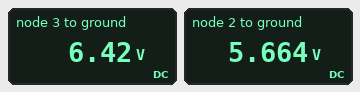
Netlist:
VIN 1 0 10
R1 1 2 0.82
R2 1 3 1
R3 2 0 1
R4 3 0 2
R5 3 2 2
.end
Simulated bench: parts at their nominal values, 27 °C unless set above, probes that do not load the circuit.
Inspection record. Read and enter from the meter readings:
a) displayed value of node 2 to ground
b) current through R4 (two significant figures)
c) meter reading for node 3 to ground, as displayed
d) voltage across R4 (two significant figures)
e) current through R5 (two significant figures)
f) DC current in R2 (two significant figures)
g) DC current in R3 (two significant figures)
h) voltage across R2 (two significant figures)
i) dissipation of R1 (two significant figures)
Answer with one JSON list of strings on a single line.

["5.664 V", "3.2 A", "6.42 V", "6.4 V", "380 mA", "3.6 A", "5.7 A", "3.6 V", "23 W"]
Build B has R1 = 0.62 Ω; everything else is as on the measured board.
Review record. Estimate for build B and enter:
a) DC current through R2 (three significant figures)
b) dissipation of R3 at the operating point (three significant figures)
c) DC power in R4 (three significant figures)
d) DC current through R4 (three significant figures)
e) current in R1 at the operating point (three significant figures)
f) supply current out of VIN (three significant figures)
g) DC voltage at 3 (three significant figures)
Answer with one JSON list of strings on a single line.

["3.44 A", "38.9 W", "21.5 W", "3.28 A", "6.07 A", "9.51 A", "6.56 V"]
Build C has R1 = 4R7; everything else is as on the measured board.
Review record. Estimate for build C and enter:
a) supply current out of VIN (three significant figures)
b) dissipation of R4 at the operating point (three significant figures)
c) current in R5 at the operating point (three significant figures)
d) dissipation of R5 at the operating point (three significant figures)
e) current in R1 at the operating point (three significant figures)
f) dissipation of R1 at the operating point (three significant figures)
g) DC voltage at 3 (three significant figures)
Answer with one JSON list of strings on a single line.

["5.78 A", "16.4 W", "1.41 A", "3.96 W", "1.51 A", "10.7 W", "5.73 V"]
